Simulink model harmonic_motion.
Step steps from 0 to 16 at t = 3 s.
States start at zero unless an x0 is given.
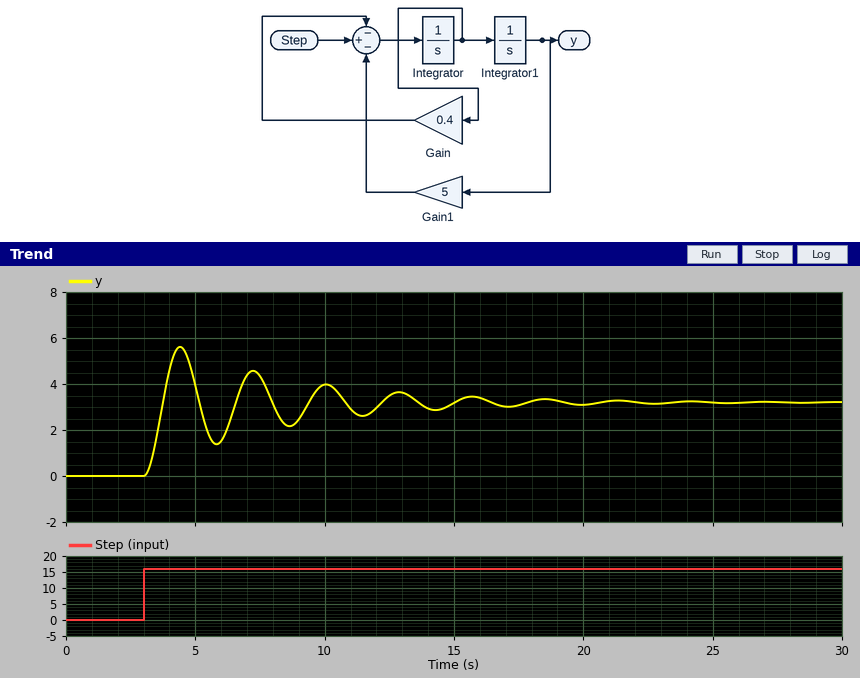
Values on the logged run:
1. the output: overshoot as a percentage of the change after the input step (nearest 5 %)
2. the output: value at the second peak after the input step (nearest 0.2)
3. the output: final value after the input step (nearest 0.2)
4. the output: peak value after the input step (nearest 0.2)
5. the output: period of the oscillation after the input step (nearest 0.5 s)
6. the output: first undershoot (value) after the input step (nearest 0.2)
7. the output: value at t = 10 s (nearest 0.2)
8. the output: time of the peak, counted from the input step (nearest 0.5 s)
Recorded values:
75 %
4.6
3.2
5.6
3.0 s
1.4
4.0
1.5 s
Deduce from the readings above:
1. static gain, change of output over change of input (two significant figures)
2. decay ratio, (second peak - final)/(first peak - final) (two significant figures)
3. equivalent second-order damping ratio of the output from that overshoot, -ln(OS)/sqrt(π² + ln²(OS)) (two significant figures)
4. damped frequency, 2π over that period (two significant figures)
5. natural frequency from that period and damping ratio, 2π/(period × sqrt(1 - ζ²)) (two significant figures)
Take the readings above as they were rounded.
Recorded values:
0.20
0.58
0.091
2.1 rad/s
2.1 rad/s
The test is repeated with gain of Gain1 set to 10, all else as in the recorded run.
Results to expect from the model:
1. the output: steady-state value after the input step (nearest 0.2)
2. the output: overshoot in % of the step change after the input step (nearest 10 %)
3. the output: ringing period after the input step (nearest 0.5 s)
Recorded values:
1.6
80 %
2.0 s
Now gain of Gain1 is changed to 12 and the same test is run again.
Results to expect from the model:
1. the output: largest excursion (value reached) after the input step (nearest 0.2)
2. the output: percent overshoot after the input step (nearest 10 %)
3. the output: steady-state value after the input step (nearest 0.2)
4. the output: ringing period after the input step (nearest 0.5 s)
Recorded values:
2.4
80 %
1.4
2.0 s
